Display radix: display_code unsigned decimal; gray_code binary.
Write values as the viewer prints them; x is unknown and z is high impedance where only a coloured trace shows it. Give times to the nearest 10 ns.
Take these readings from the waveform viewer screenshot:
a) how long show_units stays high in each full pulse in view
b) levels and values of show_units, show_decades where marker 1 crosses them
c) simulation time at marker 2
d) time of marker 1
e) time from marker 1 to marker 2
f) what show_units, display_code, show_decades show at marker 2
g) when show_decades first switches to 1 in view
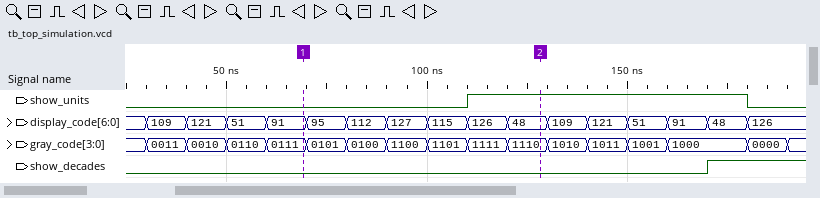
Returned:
70 ns
show_units=0, show_decades=0
130 ns
70 ns
60 ns
show_units=1, display_code=48, show_decades=0
170 ns
